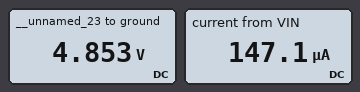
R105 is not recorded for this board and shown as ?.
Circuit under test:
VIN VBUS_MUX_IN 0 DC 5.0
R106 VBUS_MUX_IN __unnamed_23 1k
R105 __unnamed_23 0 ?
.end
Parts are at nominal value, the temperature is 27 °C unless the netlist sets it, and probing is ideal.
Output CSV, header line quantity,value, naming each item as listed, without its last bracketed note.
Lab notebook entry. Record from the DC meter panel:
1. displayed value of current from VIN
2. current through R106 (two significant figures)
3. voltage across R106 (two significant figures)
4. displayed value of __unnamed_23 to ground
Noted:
quantity,value
displayed value of current from VIN,147.1 µA
current through R106,150 µA
voltage across R106,150 mV
displayed value of __unnamed_23 to ground,4.853 V
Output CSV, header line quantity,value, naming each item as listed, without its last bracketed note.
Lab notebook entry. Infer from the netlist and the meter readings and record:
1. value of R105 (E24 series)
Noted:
quantity,value
value of R105,33 kΩ
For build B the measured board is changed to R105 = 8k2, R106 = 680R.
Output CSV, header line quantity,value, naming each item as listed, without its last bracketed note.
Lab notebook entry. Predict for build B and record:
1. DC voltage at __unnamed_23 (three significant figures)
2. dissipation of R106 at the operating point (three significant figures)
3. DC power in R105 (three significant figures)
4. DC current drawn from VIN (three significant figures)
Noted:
quantity,value
DC voltage at __unnamed_23,4.62 V
dissipation of R106 at the operating point,216 µW
DC power in R105,2.60 mW
DC current drawn from VIN,563 µA
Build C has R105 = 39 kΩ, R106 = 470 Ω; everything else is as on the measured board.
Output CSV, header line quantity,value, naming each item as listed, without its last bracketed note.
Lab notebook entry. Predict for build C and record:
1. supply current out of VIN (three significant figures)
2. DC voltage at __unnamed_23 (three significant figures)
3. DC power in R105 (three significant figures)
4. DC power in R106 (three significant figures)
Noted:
quantity,value
supply current out of VIN,127 µA
DC voltage at __unnamed_23,4.94 V
DC power in R105,626 µW
DC power in R106,7.54 µW
